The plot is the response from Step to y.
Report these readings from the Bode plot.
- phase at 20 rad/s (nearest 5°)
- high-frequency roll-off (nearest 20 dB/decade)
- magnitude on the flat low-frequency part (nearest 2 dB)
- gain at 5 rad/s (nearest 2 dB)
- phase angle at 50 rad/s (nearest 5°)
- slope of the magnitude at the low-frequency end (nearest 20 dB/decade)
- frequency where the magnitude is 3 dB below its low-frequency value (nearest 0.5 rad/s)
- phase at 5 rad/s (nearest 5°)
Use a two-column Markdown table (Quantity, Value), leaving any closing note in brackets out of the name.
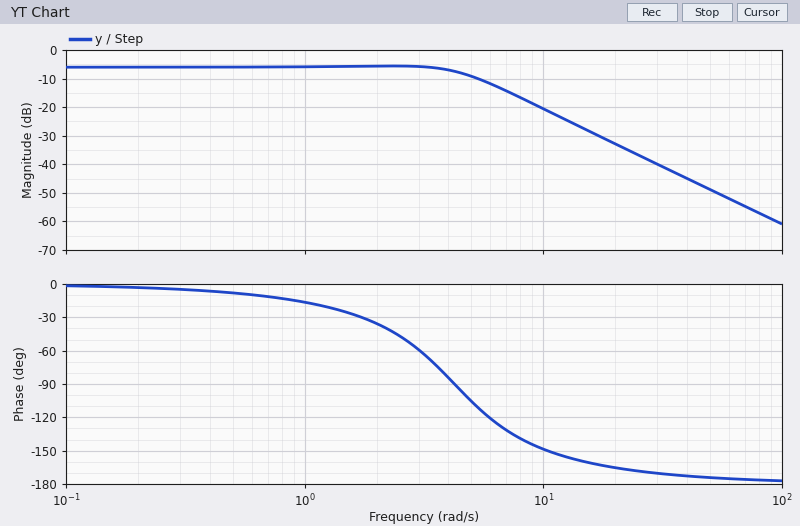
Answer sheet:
| Quantity | Value |
|---|---|
| phase at 20 rad/s | -165° |
| high-frequency roll-off | -40 dB/decade |
| magnitude on the flat low-frequency part | -6 dB |
| gain at 5 rad/s | -10 dB |
| phase angle at 50 rad/s | -175° |
| slope of the magnitude at the low-frequency end | 0 dB/decade |
| frequency where the magnitude is 3 dB below its low-frequency value | 5.0 rad/s |
| phase at 5 rad/s | -105° |
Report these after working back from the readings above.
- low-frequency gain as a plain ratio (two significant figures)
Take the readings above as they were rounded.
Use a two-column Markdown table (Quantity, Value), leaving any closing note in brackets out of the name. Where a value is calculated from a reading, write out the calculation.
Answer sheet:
| Quantity | Value |
|---|---|
| low-frequency gain as a plain ratio | 10^(-6 / 20) = 0.50 |
